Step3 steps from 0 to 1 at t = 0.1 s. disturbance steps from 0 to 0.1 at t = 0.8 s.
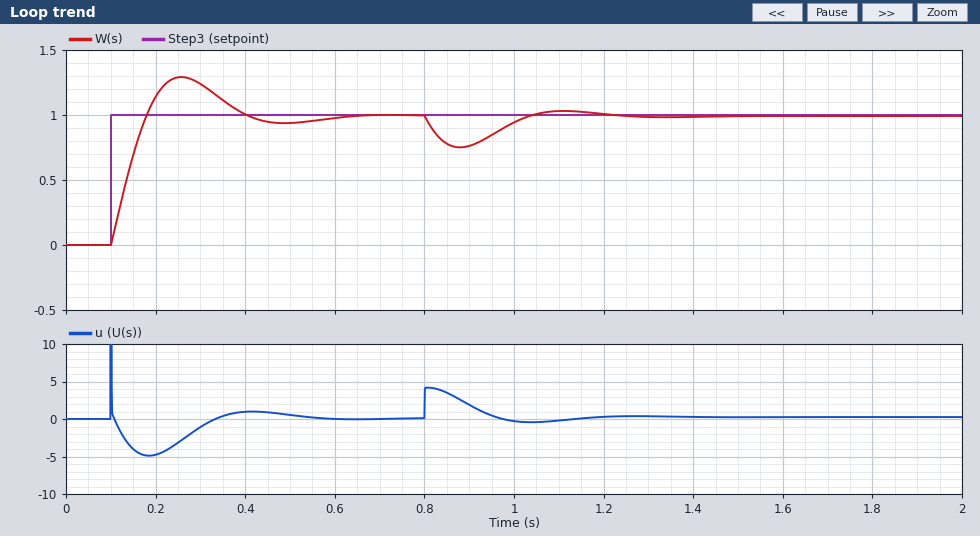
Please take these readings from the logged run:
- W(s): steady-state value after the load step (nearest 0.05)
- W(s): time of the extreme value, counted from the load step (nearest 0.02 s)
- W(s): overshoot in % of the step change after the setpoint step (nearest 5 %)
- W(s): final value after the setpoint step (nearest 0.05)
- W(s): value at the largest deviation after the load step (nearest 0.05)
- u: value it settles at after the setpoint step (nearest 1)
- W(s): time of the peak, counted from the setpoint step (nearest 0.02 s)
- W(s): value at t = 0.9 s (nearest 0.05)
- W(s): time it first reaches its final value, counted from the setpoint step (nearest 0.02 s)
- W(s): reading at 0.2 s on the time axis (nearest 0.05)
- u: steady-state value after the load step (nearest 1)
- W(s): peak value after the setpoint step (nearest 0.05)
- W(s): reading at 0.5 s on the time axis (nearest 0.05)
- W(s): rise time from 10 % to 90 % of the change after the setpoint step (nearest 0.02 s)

1.00
0.08 s
30 %
1.00
0.75
0
0.16 s
0.75
0.08 s
1.15
0
1.30
0.95
0.06 s
